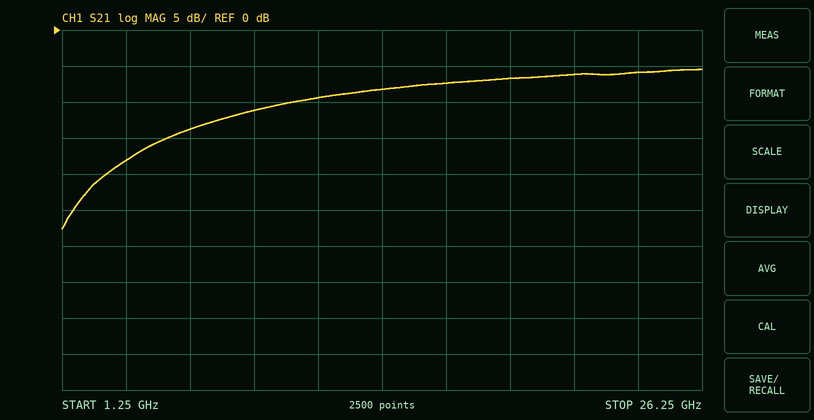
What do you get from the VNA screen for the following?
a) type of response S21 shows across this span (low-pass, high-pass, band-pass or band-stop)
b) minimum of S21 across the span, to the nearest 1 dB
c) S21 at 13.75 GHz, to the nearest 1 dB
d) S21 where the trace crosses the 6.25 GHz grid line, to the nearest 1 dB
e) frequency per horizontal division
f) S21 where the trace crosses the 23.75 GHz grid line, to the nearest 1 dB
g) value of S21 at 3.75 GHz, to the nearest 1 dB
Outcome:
high-pass
-28 dB
-8 dB
-14 dB
2.5 GHz
-6 dB
-18 dB
